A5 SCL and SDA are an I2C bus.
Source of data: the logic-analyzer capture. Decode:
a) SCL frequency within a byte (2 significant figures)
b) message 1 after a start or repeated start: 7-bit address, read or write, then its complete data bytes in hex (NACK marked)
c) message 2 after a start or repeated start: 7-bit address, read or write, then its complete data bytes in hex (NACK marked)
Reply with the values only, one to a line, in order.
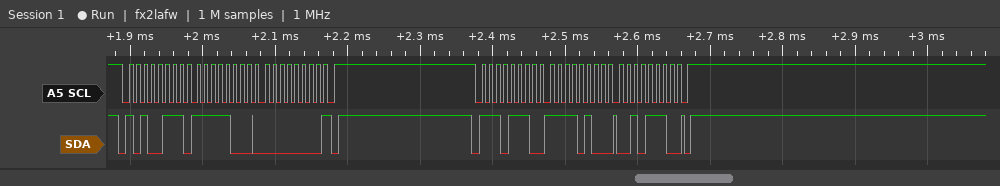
100 kHz
0x53 read: F8 00 NACK
0x77 write: F4 2E
